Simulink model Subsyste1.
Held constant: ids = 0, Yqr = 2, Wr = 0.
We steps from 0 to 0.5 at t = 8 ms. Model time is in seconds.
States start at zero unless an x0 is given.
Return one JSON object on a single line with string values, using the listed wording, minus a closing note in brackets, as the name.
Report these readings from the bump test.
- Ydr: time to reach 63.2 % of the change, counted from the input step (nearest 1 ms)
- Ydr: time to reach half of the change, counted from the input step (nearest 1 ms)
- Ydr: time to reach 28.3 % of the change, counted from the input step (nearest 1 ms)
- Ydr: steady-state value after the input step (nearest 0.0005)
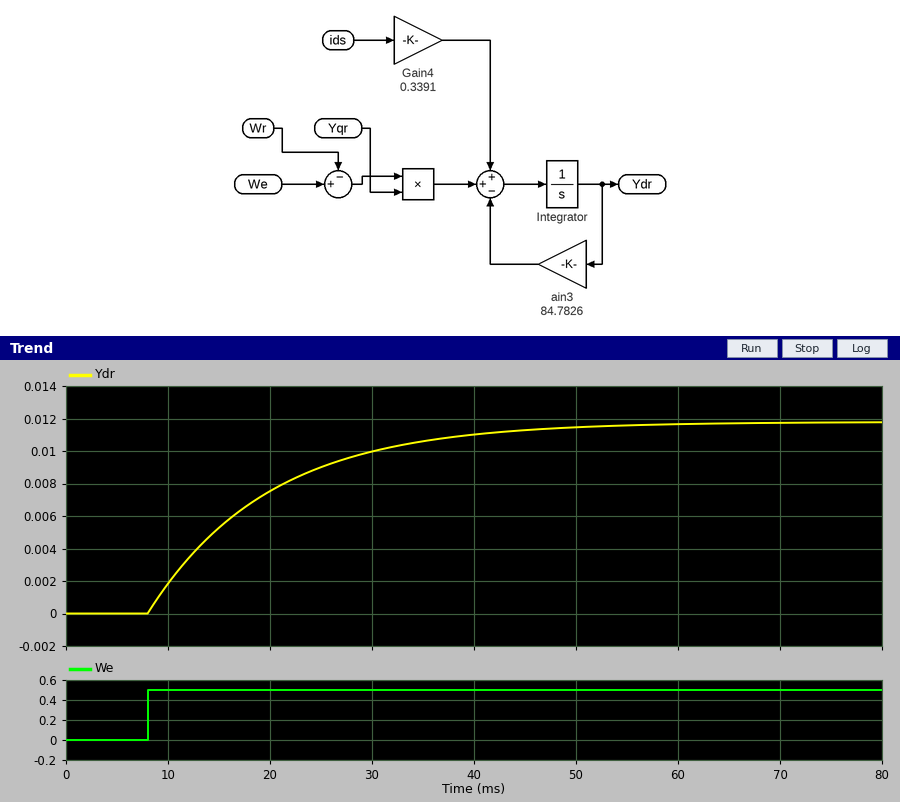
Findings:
{"Ydr: time to reach 63.2 % of the change, counted from the input step": "12 ms", "Ydr: time to reach half of the change, counted from the input step": "8 ms", "Ydr: time to reach 28.3 % of the change, counted from the input step": "4 ms", "Ydr: steady-state value after the input step": "0.0120"}
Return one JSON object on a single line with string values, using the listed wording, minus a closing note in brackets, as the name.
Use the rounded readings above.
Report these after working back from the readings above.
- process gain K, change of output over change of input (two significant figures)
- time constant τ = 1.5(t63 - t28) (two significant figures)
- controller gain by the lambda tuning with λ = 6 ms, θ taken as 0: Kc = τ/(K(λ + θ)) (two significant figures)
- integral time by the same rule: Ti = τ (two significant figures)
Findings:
{"process gain K, change of output over change of input": "0.024", "time constant τ = 1.5(t63 - t28)": "12 ms", "controller gain by the lambda tuning with λ = 6 ms, θ taken as 0: Kc = τ/(K(λ + θ))": "83", "integral time by the same rule: Ti = τ": "12 ms"}
